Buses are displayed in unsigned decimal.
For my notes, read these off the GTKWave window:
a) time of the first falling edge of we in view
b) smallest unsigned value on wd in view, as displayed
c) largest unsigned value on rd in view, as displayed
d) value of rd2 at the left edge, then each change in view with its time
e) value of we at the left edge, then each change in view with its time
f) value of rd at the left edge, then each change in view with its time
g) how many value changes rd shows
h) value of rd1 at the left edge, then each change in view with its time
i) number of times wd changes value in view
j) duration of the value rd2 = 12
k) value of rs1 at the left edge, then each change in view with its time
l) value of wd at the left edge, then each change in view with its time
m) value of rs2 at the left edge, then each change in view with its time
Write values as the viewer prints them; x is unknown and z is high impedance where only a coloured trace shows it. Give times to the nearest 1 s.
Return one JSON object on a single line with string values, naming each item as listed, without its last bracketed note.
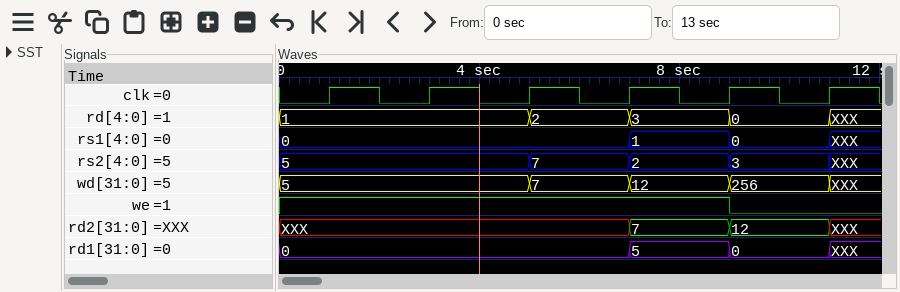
{"time of the first falling edge of we in view": "9 s", "smallest unsigned value on wd in view, as displayed": "5", "largest unsigned value on rd in view, as displayed": "3", "value of rd2 at the left edge, then each change in view with its time": "XXX, 7 at 7 s, 12 at 9 s, XXX at 11 s", "value of we at the left edge, then each change in view with its time": "1, 0 at 9 s", "value of rd at the left edge, then each change in view with its time": "1, 2 at 5 s, 3 at 7 s, 0 at 9 s, XXX at 11 s", "how many value changes rd shows": "4", "value of rd1 at the left edge, then each change in view with its time": "0, 5 at 7 s, 0 at 9 s, XXX at 11 s", "number of times wd changes value in view": "4", "duration of the value rd2 = 12": "2 s", "value of rs1 at the left edge, then each change in view with its time": "0, 1 at 7 s, 0 at 9 s, XXX at 11 s", "value of wd at the left edge, then each change in view with its time": "5, 7 at 5 s, 12 at 7 s, 256 at 9 s, XXX at 11 s", "value of rs2 at the left edge, then each change in view with its time": "5, 7 at 5 s, 2 at 7 s, 3 at 9 s, XXX at 11 s"}
